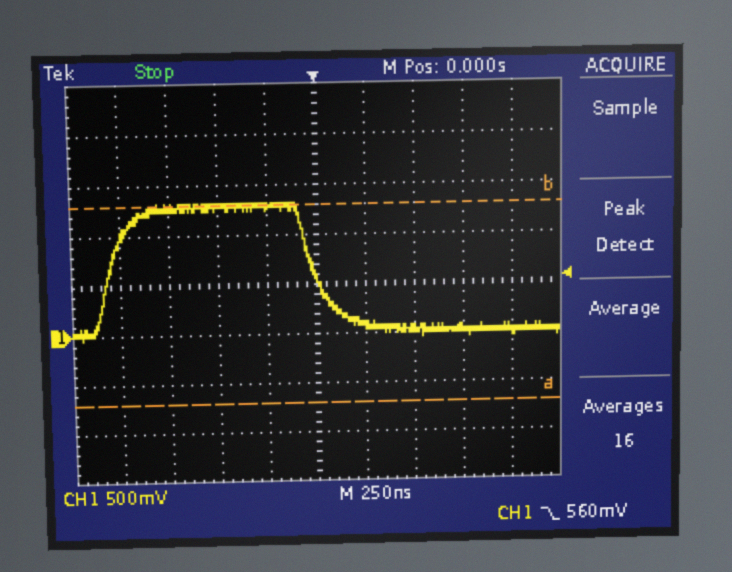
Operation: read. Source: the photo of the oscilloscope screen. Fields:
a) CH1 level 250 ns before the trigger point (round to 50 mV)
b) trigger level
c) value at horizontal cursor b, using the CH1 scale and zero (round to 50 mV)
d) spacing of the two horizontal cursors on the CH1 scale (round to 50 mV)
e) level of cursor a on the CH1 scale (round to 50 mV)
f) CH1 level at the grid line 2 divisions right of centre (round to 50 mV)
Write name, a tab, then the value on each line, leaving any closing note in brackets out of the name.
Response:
CH1 level 250 ns before the trigger point	1.30 V
trigger level	560 mV
value at horizontal cursor b, using the CH1 scale and zero	1.30 V
spacing of the two horizontal cursors on the CH1 scale	2.00 V
level of cursor a on the CH1 scale	-700 mV
CH1 level at the grid line 2 divisions right of centre	50 mV
